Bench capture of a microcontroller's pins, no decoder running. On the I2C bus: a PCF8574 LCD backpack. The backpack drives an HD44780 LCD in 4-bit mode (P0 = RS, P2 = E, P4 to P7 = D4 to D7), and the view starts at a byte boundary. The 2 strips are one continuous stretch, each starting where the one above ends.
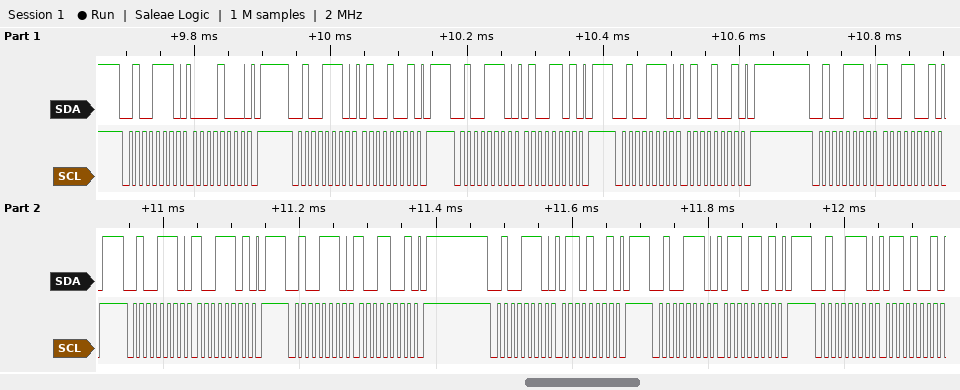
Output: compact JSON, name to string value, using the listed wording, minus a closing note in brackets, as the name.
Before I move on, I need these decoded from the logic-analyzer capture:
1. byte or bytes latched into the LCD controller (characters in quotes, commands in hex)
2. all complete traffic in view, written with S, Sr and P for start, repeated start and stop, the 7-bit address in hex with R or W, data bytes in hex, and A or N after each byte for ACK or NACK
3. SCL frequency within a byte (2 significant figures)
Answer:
{"byte or bytes latched into the LCD controller": "'I'", "all complete traffic in view, written with S, Sr and P for start, repeated start and stop, the 7-bit address in hex with R or W, data bytes in hex, and A or N after each byte for ACK or NACK": "S 27W A 08 A P S 27W A 49 A P S 27W A 4D A P S 27W A 49 A P S 27W A 99 A P S 27W A 9D A P S 27W A 99 A P S 27W A 69 A P S 27W A 6D A P S 27W A 69 A", "SCL frequency within a byte": "100 kHz"}
